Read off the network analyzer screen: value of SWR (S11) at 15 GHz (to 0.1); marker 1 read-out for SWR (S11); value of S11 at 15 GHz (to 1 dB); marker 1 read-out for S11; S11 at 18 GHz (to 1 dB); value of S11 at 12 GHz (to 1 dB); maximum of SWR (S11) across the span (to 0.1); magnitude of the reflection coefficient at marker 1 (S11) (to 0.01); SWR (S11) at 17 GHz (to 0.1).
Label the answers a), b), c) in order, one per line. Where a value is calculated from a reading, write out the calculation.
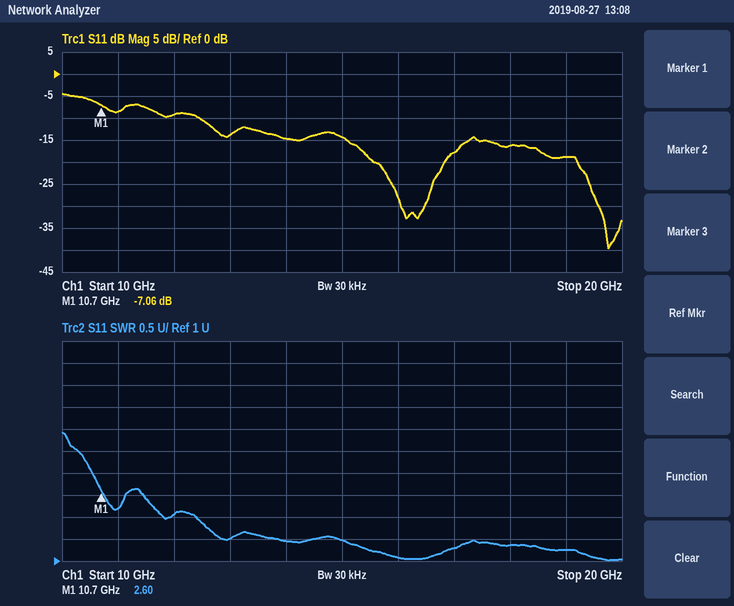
a) 1.5
b) 2.60
c) -14 dB
d) -7.06 dB
e) -16 dB
f) -9 dB
g) 3.9
h) 10^(-7.06/20) ≈ 0.44
i) 1.3
